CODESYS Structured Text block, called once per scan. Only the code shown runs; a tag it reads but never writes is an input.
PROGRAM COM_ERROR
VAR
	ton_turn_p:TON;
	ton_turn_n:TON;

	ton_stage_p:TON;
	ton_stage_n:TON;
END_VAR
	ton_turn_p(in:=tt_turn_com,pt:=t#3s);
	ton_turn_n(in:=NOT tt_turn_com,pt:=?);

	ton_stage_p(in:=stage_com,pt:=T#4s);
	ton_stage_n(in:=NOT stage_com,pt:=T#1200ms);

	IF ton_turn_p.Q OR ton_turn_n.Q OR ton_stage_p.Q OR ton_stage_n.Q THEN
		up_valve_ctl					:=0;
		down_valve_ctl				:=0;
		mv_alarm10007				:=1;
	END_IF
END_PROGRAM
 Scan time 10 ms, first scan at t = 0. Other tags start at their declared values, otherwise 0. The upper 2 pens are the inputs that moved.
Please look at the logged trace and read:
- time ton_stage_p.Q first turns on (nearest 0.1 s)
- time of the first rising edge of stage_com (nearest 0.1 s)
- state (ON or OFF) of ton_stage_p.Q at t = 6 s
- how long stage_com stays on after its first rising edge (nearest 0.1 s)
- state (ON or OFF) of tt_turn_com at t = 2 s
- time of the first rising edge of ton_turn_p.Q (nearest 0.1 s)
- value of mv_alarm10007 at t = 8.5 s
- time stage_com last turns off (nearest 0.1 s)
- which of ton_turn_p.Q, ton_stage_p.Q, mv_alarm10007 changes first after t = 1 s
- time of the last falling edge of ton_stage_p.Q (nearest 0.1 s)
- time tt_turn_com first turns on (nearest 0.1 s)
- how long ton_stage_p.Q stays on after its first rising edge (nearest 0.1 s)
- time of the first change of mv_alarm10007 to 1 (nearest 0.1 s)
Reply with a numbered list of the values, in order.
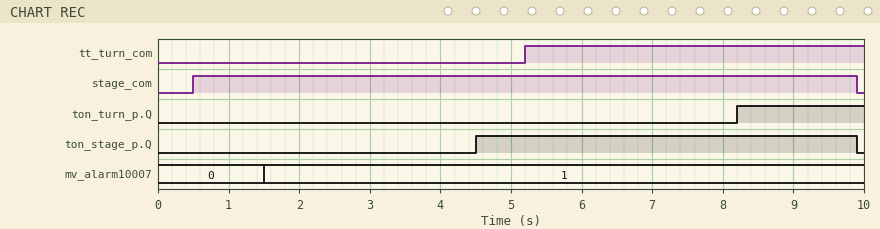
1. 4.5 s
2. 0.5 s
3. ON
4. 9.4 s
5. OFF
6. 8.2 s
7. 1
8. 9.9 s
9. mv_alarm10007
10. 9.9 s
11. 5.2 s
12. 5.4 s
13. 1.5 s
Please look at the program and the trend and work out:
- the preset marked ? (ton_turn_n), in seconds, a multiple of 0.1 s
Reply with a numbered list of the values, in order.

1. 1.5 s
